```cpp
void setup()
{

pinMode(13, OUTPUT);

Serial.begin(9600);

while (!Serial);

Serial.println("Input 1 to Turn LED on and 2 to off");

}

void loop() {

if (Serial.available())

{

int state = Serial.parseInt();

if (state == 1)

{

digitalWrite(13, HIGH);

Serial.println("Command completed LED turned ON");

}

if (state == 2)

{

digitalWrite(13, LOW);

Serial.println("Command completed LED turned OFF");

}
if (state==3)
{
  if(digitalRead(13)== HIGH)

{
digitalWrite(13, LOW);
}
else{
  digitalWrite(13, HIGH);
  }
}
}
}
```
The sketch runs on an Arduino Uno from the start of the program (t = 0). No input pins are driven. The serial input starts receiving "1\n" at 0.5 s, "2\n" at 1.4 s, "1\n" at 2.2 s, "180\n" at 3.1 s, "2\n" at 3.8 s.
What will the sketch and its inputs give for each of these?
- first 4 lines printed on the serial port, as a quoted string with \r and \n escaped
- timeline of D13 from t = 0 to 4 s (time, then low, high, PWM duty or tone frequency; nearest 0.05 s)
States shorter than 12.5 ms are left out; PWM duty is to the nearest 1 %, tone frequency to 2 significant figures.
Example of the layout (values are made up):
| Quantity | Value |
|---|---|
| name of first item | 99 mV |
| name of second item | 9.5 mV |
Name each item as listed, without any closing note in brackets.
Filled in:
| Quantity | Value |
|---|---|
| first 4 lines printed on the serial port, as a quoted string with \r and \n escaped | "Input 1 to Turn LED on and 2 to off\r\nCommand completed LED turned ON\r\nCommand completed LED turned OFF\r\nCommand completed LED turned ON\r\n" |
| timeline of D13 from t = 0 to 4 s | 0 s low; 0.5 s high; 1.4 s low; 2.2 s high; 3.8 s low |
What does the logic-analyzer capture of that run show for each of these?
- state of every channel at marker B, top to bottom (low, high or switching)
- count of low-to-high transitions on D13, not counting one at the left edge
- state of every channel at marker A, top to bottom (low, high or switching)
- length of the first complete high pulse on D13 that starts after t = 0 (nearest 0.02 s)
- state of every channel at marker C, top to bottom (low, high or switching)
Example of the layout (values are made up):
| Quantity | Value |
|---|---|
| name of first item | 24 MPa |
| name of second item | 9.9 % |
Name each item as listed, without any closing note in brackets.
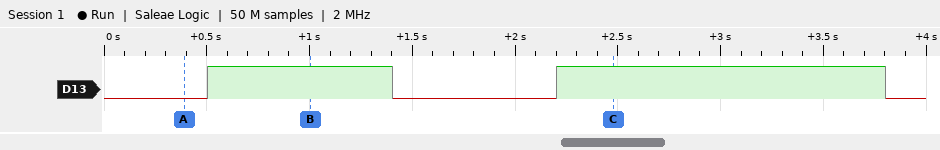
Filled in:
| Quantity | Value |
|---|---|
| state of every channel at marker B, top to bottom | D13 high |
| count of low-to-high transitions on D13, not counting one at the left edge | 2 |
| state of every channel at marker A, top to bottom | D13 low |
| length of the first complete high pulse on D13 that starts after t = 0 | 0.90 s |
| state of every channel at marker C, top to bottom | D13 high |
